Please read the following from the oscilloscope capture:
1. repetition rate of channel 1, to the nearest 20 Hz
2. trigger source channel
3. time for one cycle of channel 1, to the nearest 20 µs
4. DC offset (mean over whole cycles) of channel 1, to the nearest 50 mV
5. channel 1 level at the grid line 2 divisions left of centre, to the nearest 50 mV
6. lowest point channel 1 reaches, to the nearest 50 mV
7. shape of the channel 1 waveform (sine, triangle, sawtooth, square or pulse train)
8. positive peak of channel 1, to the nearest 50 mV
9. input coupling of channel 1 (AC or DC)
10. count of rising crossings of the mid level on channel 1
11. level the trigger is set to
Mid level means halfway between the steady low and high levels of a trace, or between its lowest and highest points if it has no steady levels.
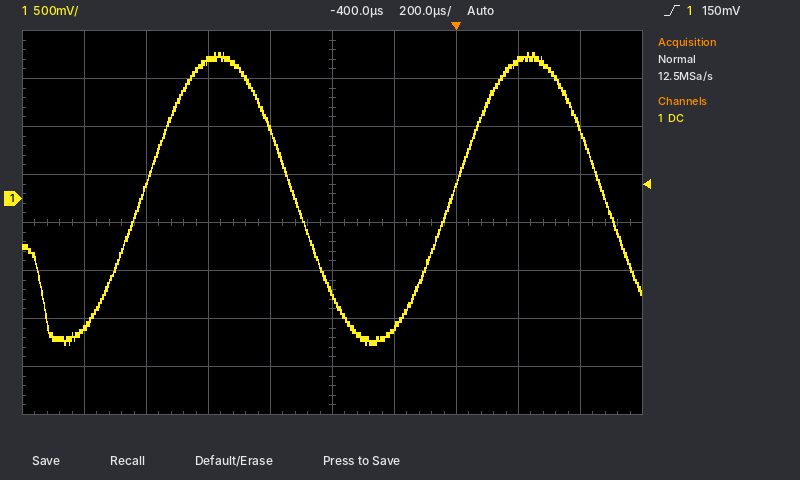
1.00 kHz
channel 1
1.00 ms
0 mV
1.45 V
-1.50 V
sine
1.50 V
DC
2
150 mV
